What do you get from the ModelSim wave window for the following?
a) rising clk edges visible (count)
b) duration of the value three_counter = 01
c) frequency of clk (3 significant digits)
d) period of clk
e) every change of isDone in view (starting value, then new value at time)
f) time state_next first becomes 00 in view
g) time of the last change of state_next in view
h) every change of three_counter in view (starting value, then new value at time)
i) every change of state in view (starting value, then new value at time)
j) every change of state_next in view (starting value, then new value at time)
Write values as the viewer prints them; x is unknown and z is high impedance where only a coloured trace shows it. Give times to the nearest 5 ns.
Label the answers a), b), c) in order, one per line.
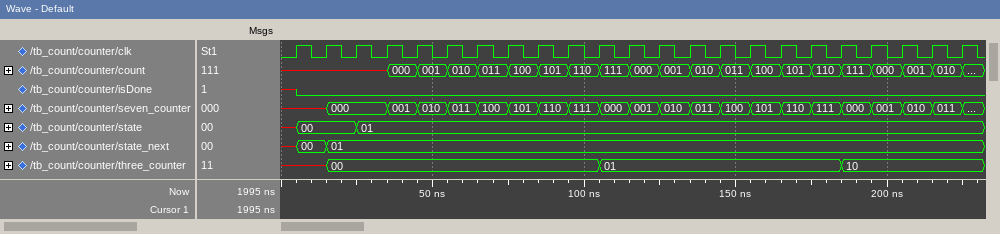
a) 23
b) 80 ns
c) 100 MHz
d) 10 ns
e) x, 0 at 5 ns
f) 5 ns
g) 15 ns
h) x, 00 at 15 ns, 01 at 105 ns, 10 at 185 ns
i) x, 00 at 5 ns, 01 at 25 ns
j) x, 00 at 5 ns, 01 at 15 ns
